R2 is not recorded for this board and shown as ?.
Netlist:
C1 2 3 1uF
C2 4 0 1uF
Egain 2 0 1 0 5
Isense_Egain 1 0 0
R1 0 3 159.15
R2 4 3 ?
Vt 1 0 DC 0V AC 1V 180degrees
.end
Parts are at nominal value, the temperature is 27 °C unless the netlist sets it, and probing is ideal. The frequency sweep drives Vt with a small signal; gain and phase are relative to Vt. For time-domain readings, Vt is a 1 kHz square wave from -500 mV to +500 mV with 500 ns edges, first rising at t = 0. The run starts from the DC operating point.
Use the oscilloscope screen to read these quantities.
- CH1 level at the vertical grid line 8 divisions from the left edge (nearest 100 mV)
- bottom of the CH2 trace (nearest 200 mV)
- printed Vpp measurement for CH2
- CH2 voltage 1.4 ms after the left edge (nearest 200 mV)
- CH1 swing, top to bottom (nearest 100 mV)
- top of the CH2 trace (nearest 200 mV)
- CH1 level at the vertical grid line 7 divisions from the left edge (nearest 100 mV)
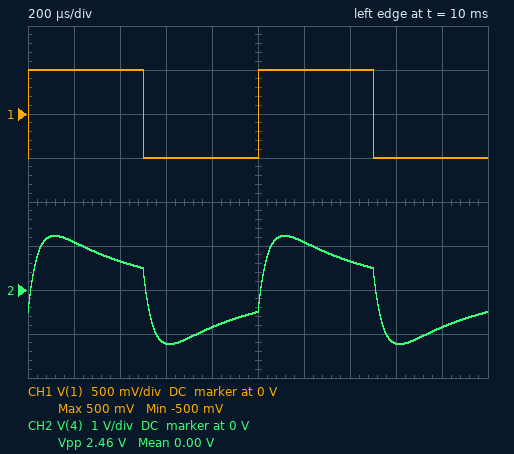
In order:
-500 mV
-1.2 V
2.46 V
600 mV
1.0 V
1.2 V
500 mV
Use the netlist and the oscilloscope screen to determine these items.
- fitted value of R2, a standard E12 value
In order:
100 Ω
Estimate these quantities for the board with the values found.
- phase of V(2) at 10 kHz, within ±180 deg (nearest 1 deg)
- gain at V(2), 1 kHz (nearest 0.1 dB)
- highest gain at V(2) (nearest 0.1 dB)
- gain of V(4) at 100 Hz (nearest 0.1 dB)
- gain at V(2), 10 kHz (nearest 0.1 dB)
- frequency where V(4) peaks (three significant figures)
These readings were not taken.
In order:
0 deg
14.0 dB
14.0 dB
-6.3 dB
14.0 dB
1.26 kHz
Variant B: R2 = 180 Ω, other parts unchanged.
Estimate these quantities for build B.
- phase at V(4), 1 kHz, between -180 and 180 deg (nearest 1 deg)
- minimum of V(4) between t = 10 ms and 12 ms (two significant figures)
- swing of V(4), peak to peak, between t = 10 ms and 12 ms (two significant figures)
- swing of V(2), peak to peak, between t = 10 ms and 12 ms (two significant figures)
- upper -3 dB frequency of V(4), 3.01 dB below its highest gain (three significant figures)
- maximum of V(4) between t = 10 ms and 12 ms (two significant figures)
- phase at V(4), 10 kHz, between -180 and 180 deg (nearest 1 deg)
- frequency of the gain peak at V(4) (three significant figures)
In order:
-2 deg
-950 mV
1.9 V
5.0 V
3.06 kHz
950 mV
-74 deg
940 Hz
